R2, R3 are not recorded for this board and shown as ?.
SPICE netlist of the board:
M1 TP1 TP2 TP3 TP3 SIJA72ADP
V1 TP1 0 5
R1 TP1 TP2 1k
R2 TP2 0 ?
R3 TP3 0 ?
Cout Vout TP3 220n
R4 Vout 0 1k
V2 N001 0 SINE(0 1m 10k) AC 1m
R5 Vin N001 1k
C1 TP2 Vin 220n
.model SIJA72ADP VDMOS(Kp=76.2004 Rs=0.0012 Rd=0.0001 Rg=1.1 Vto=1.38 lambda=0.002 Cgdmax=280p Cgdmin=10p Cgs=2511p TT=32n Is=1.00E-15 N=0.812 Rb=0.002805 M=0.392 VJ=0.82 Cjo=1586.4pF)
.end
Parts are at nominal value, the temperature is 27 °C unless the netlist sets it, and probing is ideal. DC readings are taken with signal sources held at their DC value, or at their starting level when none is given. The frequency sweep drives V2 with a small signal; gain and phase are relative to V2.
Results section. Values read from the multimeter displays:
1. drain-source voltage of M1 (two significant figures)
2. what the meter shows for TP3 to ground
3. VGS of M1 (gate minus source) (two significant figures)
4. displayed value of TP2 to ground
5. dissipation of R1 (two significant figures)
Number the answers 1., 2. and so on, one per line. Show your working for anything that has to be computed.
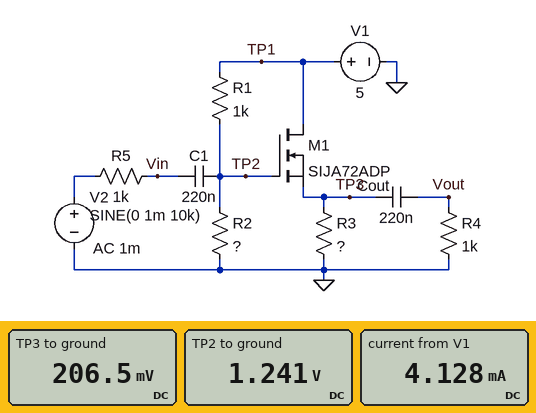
1. 5 V - 206.5 mV = 4.8 V
2. 206.5 mV
3. 1.241 V - 206.5 mV = 1.0 V
4. 1.241 V
5. (5 V - 1.241 V)^2 / 1 kΩ = 14 mW
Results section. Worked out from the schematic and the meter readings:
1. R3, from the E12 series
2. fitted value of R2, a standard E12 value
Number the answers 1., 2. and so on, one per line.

1. 560 Ω
2. 330 Ω
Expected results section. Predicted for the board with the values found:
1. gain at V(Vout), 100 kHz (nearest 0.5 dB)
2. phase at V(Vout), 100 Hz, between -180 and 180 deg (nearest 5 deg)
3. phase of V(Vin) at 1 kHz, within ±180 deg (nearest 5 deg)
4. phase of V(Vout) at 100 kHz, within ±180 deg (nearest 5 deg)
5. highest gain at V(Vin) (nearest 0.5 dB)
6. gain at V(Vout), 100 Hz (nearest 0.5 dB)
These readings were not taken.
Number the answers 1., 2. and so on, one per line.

1. -17.0 dB
2. 160 deg
3. -40 deg
4. -5 deg
5. 0 dB
6. -48.5 dB
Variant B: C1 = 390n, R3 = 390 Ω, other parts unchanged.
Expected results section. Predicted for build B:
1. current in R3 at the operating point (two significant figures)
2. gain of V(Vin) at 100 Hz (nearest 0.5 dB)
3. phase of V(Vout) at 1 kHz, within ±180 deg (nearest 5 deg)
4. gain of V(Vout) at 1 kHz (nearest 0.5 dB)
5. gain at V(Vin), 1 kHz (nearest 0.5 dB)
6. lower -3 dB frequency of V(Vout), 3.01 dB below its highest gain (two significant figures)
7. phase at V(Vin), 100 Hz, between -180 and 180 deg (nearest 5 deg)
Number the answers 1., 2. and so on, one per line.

1. 490 µA
2. -0.5 dB
3. 50 deg
4. -19.0 dB
5. -9.0 dB
6. 790 Hz
7. -15 deg
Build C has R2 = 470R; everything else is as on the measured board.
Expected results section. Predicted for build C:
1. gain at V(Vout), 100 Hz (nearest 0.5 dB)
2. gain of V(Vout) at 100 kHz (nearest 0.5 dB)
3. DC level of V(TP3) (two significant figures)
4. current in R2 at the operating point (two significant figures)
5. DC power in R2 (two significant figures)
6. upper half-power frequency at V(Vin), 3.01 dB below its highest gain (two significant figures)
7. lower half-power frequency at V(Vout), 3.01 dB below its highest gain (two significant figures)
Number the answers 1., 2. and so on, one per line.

1. -45.5 dB
2. -13.5 dB
3. 520 mV
4. 3.4 mA
5. 5.4 mW
6. 580 Hz
7. 970 Hz
